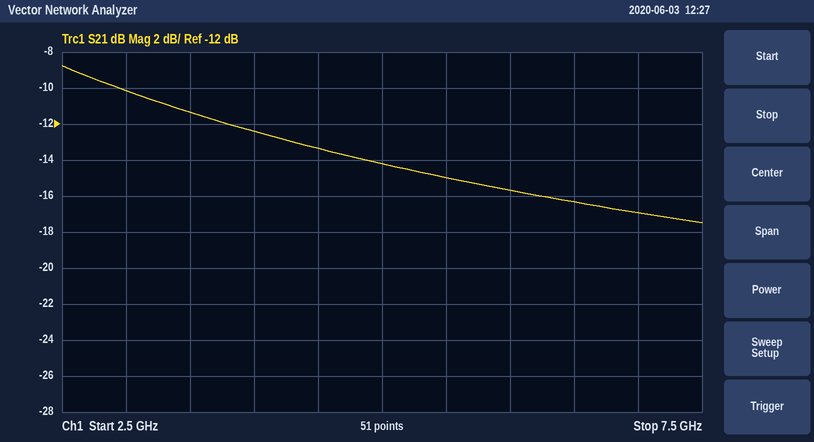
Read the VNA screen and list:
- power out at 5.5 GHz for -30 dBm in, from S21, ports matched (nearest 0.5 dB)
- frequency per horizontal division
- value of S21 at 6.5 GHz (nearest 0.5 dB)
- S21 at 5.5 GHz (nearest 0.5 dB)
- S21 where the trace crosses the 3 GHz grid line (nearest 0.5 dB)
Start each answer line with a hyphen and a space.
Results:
- -45.0 dBm
- 500 MHz
- -16.5 dB
- -15.0 dB
- -10.0 dB
